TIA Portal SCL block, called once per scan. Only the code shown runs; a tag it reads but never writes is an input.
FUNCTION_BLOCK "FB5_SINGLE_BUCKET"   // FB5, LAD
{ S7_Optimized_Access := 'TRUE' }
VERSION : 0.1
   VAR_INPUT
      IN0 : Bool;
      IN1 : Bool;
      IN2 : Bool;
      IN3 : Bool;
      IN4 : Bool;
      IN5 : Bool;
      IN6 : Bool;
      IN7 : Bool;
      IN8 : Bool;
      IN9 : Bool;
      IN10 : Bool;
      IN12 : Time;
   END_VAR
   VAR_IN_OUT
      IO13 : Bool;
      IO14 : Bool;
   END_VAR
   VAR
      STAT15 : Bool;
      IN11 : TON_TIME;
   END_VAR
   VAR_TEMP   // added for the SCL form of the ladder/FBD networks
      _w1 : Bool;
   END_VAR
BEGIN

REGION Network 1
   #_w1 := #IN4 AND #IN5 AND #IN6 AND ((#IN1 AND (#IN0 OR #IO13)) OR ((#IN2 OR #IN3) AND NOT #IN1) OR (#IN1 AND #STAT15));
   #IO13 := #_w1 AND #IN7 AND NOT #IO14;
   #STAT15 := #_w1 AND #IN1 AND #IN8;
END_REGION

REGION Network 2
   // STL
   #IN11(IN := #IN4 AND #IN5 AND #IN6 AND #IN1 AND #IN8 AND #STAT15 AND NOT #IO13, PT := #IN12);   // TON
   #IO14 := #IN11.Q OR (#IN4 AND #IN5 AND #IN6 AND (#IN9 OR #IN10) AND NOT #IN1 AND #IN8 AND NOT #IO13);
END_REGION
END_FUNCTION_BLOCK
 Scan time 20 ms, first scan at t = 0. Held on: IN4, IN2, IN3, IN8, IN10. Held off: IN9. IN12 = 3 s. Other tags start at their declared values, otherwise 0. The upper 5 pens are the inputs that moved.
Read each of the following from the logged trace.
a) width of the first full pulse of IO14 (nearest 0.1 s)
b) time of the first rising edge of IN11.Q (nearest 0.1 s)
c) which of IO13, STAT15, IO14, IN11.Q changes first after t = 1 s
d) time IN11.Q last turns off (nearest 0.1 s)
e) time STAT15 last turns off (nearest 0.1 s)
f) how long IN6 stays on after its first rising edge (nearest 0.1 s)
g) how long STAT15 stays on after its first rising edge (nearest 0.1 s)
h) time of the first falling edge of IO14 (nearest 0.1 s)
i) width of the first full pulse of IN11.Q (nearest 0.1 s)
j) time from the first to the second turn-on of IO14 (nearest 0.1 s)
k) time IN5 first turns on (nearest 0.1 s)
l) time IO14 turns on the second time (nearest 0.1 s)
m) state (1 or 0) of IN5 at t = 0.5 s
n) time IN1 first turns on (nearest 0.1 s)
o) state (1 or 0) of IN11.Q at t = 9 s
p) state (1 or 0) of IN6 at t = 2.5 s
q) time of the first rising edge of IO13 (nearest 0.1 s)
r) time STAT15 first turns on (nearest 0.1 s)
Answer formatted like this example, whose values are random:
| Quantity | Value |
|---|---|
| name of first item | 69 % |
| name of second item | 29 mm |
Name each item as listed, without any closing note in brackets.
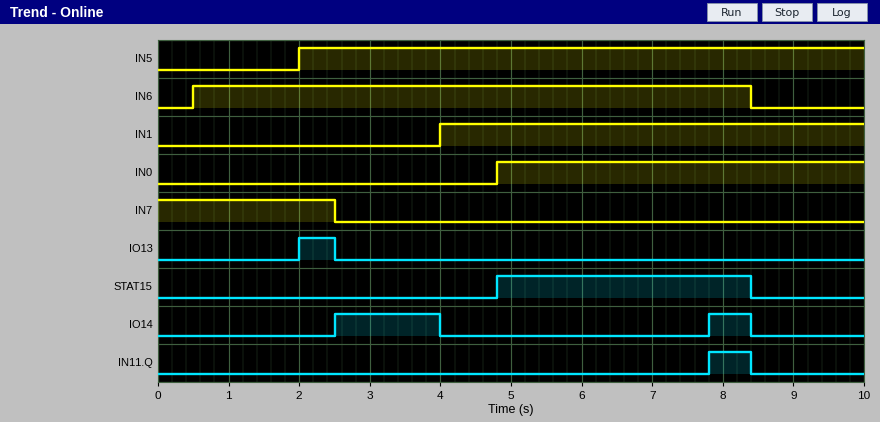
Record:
| Quantity | Value |
|---|---|
| width of the first full pulse of IO14 | 1.5 s |
| time of the first rising edge of IN11.Q | 7.8 s |
| which of IO13, STAT15, IO14, IN11.Q changes first after t = 1 s | IO13 |
| time IN11.Q last turns off | 8.4 s |
| time STAT15 last turns off | 8.4 s |
| how long IN6 stays on after its first rising edge | 7.9 s |
| how long STAT15 stays on after its first rising edge | 3.6 s |
| time of the first falling edge of IO14 | 4.0 s |
| width of the first full pulse of IN11.Q | 0.6 s |
| time from the first to the second turn-on of IO14 | 5.3 s |
| time IN5 first turns on | 2.0 s |
| time IO14 turns on the second time | 7.8 s |
| state (1 or 0) of IN5 at t = 0.5 s | 0 |
| time IN1 first turns on | 4.0 s |
| state (1 or 0) of IN11.Q at t = 9 s | 0 |
| state (1 or 0) of IN6 at t = 2.5 s | 1 |
| time of the first rising edge of IO13 | 2.0 s |
| time STAT15 first turns on | 4.8 s |
